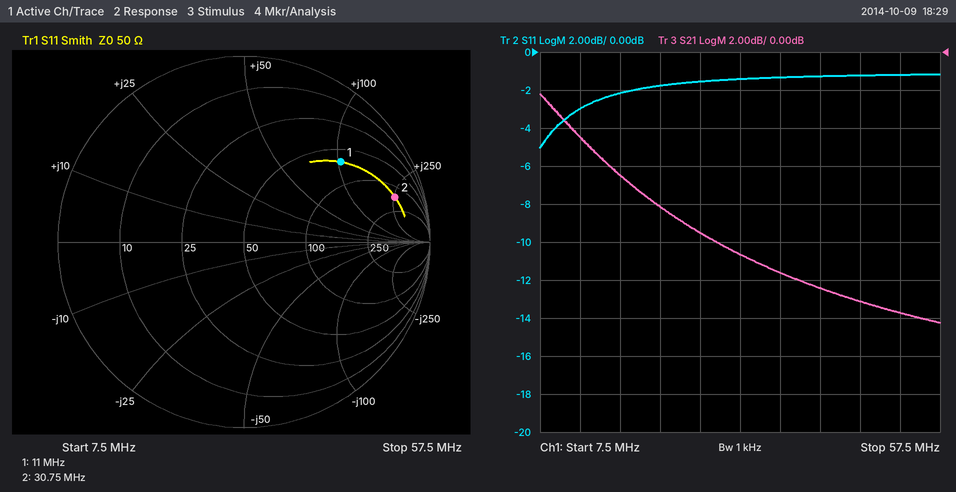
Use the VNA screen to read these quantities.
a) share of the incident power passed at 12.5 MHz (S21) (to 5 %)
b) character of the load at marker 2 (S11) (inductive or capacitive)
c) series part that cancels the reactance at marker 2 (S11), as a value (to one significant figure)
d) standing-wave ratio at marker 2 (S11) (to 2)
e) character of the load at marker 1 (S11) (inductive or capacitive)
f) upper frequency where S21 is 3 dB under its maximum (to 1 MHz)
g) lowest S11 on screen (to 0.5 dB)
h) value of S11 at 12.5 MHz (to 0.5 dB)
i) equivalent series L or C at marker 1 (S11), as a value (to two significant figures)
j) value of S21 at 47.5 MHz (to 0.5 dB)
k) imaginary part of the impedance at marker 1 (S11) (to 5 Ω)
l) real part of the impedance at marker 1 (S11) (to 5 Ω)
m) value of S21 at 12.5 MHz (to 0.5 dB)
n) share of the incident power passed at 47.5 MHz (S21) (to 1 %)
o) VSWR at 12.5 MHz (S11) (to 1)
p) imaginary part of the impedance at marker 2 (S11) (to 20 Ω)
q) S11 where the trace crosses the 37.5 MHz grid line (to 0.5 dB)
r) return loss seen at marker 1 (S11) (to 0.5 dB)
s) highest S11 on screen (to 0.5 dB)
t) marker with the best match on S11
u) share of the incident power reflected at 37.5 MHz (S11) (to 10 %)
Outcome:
35 %
inductive
20 pF
12
inductive
14 MHz
-5.0 dB
-3.0 dB
1.5 µH
-13.0 dB
+105 Ω
65 Ω
-4.5 dB
5 %
6
+260 Ω
-1.5 dB
3.5 dB
-1.0 dB
marker 1
70 %
